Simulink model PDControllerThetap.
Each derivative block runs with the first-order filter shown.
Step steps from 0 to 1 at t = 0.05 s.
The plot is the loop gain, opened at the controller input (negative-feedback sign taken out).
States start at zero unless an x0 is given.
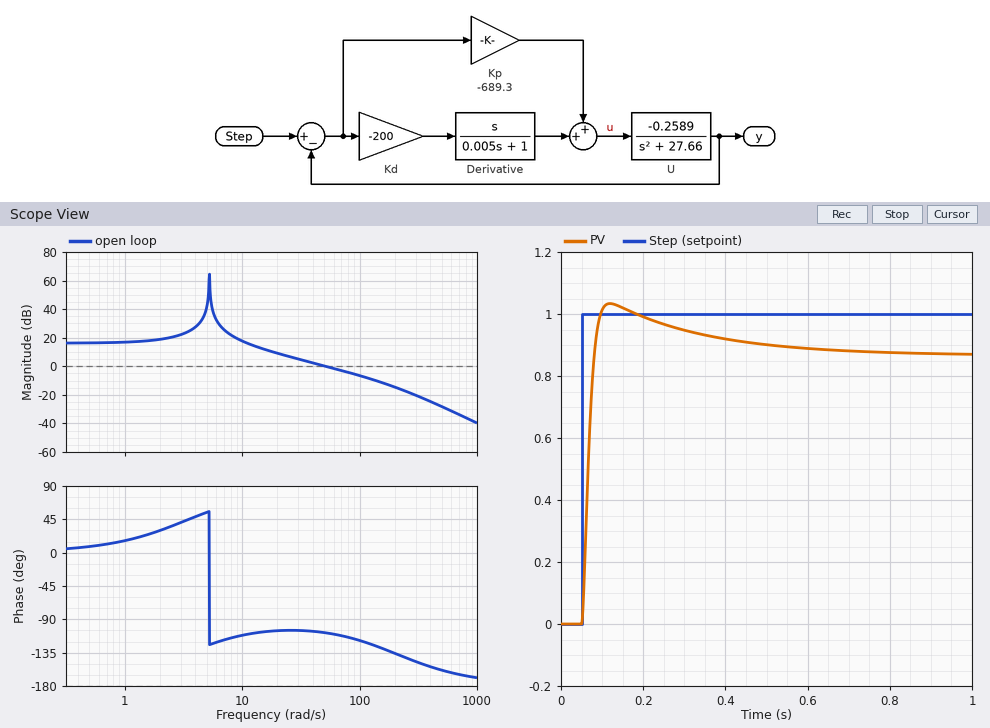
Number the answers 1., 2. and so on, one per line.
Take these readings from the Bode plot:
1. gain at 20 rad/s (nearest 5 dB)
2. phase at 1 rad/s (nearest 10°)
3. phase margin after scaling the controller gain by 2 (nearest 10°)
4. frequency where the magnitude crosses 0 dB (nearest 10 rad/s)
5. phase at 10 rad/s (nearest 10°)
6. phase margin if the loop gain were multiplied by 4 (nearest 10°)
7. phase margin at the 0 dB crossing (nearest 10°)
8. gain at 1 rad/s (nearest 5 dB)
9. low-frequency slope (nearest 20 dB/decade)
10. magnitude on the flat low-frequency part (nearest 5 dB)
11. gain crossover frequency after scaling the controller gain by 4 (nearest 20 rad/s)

1. 10 dB
2. 20°
3. 60°
4. 50 rad/s
5. -110°
6. 50°
7. 70°
8. 15 dB
9. 0 dB/decade
10. 15 dB
11. 160 rad/s
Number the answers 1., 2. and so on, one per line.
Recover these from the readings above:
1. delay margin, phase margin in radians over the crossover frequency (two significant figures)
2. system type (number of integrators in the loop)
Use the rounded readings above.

1. 0.024 s
2. 0
